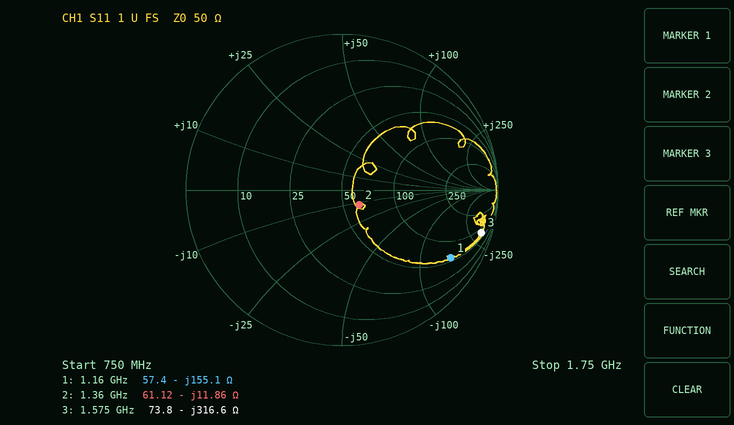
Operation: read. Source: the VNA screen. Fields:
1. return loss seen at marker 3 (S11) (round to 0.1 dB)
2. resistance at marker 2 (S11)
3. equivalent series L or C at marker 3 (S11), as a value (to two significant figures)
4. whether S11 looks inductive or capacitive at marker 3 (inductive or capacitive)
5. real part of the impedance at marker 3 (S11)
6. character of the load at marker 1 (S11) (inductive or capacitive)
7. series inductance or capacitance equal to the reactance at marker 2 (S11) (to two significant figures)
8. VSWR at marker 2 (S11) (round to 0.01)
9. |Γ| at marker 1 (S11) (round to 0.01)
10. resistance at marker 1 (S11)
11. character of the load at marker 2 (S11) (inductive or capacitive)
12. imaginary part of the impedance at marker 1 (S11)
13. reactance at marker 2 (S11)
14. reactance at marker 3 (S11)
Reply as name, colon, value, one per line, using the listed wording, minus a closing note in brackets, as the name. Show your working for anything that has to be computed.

return loss seen at marker 3 (S11): 0.6 dB
resistance at marker 2: 61.12 Ω
equivalent series L or C at marker 3 (S11), as a value: C = 1/(2π × 1.575 GHz × 316.6 Ω) ≈ 319 fF, so 320 fF to two significant figures
whether S11 looks inductive or capacitive at marker 3: capacitive
real part of the impedance at marker 3: 73.8 Ω
character of the load at marker 1 (S11): capacitive
series inductance or capacitance equal to the reactance at marker 2 (S11): C = 1/(2π × 1.36 GHz × 11.86 Ω) ≈ 9.9 pF
VSWR at marker 2 (S11): 1.34
|Γ| at marker 1 (S11): 0.82
resistance at marker 1: 57.4 Ω
character of the load at marker 2 (S11): capacitive
imaginary part of the impedance at marker 1: -155.1 Ω
reactance at marker 2: -11.86 Ω
reactance at marker 3: -316.6 Ω
